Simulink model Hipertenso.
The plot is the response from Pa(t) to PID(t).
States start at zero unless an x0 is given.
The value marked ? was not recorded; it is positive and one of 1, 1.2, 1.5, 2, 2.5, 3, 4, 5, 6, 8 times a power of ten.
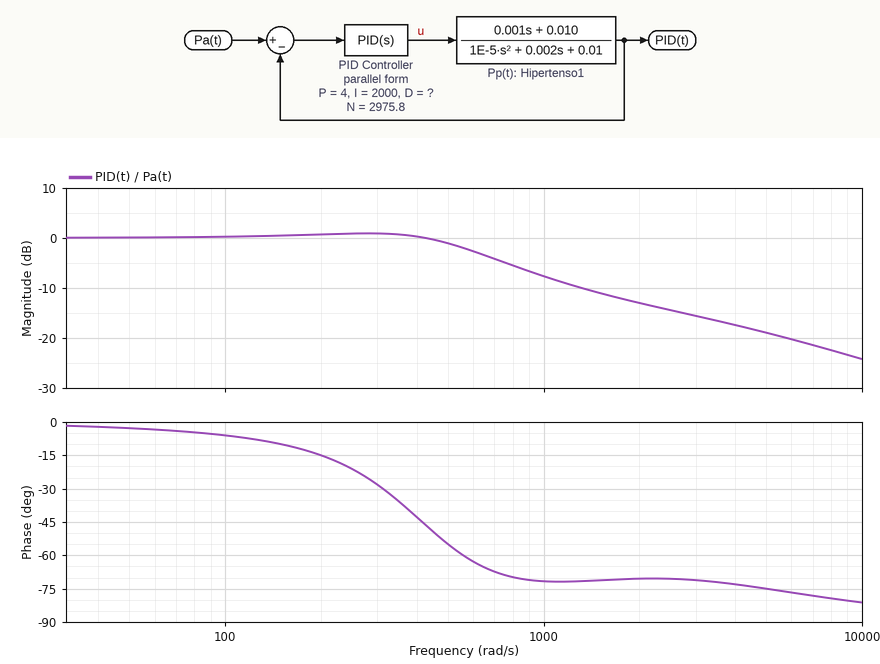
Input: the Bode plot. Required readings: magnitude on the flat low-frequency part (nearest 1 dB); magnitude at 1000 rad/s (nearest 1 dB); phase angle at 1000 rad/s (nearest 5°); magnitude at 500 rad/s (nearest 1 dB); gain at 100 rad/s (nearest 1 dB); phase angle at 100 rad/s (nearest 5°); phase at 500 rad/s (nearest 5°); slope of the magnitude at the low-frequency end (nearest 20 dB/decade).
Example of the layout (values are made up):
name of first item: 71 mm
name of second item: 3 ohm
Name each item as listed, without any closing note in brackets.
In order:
magnitude on the flat low-frequency part: 0 dB
magnitude at 1000 rad/s: -8 dB
phase angle at 1000 rad/s: -70°
magnitude at 500 rad/s: -1 dB
gain at 100 rad/s: 0 dB
phase angle at 100 rad/s: -5°
phase at 500 rad/s: -55°
slope of the magnitude at the low-frequency end: 0 dB/decade
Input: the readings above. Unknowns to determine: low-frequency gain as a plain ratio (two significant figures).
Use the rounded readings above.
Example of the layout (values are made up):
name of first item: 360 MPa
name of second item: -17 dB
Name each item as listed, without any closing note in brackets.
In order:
low-frequency gain as a plain ratio: 1.0
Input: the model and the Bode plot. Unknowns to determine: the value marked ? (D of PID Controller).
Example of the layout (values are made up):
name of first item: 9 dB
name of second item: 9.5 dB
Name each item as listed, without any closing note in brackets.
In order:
the value marked ?: 0.0008
